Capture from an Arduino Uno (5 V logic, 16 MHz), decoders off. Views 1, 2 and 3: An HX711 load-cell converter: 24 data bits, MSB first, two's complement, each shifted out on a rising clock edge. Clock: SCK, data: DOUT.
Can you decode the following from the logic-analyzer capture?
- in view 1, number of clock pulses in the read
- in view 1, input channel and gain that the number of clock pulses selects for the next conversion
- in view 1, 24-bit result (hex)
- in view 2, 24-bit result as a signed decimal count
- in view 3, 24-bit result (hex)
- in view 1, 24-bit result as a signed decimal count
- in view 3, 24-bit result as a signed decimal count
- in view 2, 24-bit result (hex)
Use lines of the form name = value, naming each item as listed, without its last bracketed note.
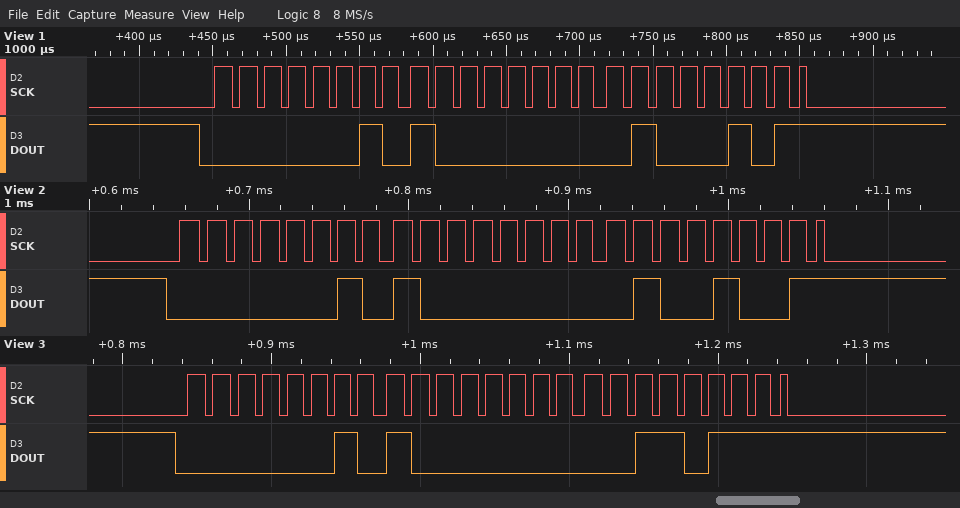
in view 1, number of clock pulses in the read = 25
in view 1, input channel and gain that the number of clock pulses selects for the next conversion = channel A, gain 128
in view 1, 24-bit result = 0x028045
in view 2, 24-bit result as a signed decimal count = 163913
in view 3, 24-bit result = 0x028037
in view 1, 24-bit result as a signed decimal count = 163909
in view 3, 24-bit result as a signed decimal count = 163895
in view 2, 24-bit result = 0x028049
